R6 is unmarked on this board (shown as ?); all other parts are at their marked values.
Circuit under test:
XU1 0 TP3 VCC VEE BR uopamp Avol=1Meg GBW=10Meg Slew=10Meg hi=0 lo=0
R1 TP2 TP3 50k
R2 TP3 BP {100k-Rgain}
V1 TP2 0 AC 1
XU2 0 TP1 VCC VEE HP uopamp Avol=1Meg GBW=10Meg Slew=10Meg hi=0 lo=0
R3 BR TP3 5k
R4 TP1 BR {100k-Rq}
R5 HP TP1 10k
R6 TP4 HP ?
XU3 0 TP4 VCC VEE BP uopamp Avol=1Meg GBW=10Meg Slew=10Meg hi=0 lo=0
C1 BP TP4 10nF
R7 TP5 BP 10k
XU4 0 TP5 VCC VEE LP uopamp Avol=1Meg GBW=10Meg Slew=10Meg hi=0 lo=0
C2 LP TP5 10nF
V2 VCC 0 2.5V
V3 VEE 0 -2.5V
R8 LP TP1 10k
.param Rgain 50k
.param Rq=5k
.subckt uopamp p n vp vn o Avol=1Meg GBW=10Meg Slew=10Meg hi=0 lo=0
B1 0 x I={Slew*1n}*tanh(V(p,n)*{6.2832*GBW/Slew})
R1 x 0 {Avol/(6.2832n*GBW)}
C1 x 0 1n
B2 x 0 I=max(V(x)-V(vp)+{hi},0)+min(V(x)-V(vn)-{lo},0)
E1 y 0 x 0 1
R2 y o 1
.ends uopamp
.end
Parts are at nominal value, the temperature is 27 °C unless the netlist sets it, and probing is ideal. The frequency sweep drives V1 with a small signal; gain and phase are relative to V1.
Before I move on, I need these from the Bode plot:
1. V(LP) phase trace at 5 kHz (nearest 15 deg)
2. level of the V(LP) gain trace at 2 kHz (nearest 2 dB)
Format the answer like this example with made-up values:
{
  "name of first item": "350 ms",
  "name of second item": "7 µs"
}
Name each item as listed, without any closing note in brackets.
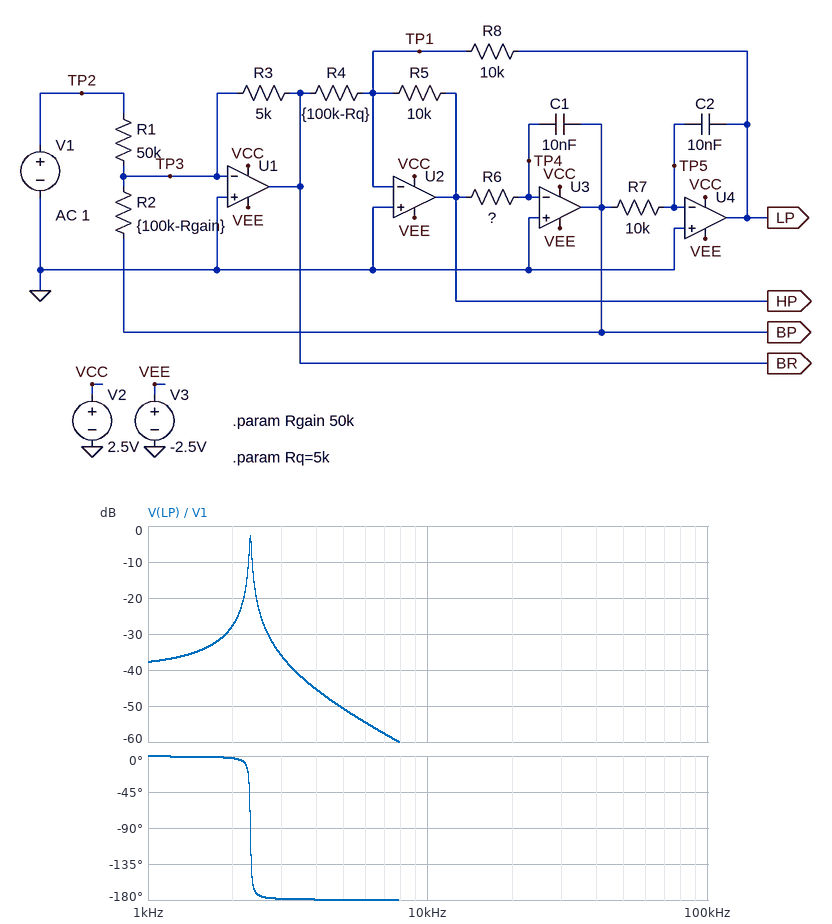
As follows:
{
  "V(LP) phase trace at 5 kHz": "-180 deg",
  "level of the V(LP) gain trace at 2 kHz": "-28 dB"
}
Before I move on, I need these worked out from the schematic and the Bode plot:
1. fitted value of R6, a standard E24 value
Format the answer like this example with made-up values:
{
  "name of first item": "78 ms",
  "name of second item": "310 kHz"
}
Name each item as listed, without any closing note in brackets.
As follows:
{
  "fitted value of R6, a standard E24 value": "4.7 kΩ"
}
